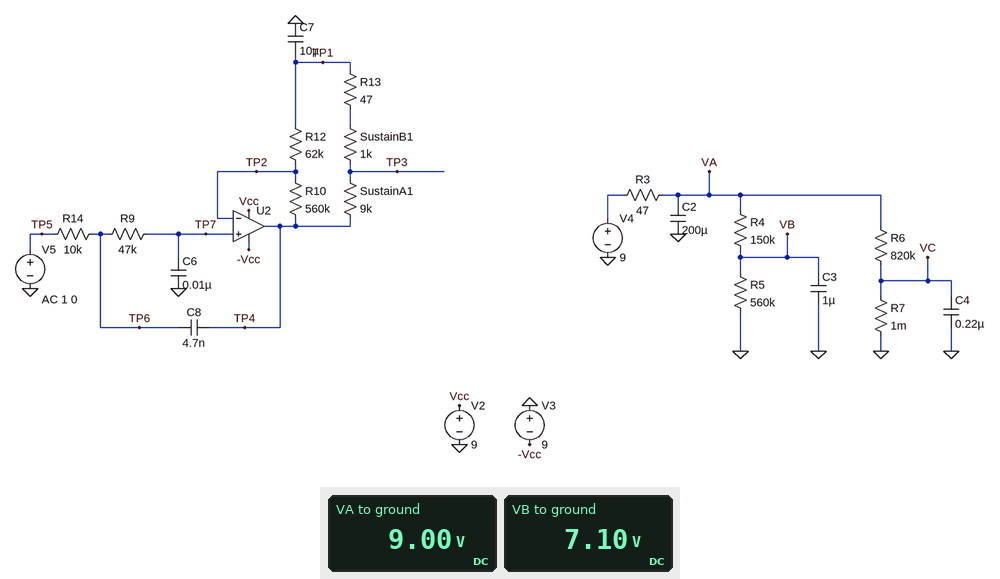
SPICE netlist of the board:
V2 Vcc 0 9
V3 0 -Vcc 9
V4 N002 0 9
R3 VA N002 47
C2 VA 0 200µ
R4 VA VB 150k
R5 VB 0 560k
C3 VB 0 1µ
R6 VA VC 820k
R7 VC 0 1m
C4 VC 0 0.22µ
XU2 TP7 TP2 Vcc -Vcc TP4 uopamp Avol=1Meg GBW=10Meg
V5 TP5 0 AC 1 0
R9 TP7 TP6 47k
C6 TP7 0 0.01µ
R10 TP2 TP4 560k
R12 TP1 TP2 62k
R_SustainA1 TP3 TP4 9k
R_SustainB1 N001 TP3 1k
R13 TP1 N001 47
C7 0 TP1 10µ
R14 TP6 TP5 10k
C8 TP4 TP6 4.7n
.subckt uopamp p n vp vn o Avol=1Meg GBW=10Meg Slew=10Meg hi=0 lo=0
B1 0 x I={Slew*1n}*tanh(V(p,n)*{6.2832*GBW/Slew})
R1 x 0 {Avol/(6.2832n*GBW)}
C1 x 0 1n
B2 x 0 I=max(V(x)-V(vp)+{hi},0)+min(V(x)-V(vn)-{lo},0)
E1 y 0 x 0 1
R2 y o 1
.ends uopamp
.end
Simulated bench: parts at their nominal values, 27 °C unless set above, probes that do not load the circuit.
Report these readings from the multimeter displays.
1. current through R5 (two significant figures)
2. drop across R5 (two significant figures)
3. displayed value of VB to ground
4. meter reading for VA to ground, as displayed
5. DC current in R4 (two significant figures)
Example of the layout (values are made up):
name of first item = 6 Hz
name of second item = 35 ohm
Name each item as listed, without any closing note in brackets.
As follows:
current through R5 = 13 µA
drop across R5 = 7.1 V
displayed value of VB to ground = 7.10 V
meter reading for VA to ground, as displayed = 9.00 V
DC current in R4 = 13 µA
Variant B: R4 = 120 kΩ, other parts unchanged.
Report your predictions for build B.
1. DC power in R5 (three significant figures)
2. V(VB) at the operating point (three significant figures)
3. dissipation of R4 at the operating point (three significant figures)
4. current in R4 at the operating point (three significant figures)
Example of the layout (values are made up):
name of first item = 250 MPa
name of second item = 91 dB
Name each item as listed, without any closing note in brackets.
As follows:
DC power in R5 = 98.1 µW
V(VB) at the operating point = 7.41 V
dissipation of R4 at the operating point = 21.0 µW
current in R4 at the operating point = 13.2 µA
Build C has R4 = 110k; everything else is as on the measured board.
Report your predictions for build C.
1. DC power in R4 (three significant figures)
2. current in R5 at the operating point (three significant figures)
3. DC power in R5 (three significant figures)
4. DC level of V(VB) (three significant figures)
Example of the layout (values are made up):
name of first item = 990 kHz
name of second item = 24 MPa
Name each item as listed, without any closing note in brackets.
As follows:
DC power in R4 = 19.8 µW
current in R5 at the operating point = 13.4 µA
DC power in R5 = 101 µW
DC level of V(VB) = 7.52 V
